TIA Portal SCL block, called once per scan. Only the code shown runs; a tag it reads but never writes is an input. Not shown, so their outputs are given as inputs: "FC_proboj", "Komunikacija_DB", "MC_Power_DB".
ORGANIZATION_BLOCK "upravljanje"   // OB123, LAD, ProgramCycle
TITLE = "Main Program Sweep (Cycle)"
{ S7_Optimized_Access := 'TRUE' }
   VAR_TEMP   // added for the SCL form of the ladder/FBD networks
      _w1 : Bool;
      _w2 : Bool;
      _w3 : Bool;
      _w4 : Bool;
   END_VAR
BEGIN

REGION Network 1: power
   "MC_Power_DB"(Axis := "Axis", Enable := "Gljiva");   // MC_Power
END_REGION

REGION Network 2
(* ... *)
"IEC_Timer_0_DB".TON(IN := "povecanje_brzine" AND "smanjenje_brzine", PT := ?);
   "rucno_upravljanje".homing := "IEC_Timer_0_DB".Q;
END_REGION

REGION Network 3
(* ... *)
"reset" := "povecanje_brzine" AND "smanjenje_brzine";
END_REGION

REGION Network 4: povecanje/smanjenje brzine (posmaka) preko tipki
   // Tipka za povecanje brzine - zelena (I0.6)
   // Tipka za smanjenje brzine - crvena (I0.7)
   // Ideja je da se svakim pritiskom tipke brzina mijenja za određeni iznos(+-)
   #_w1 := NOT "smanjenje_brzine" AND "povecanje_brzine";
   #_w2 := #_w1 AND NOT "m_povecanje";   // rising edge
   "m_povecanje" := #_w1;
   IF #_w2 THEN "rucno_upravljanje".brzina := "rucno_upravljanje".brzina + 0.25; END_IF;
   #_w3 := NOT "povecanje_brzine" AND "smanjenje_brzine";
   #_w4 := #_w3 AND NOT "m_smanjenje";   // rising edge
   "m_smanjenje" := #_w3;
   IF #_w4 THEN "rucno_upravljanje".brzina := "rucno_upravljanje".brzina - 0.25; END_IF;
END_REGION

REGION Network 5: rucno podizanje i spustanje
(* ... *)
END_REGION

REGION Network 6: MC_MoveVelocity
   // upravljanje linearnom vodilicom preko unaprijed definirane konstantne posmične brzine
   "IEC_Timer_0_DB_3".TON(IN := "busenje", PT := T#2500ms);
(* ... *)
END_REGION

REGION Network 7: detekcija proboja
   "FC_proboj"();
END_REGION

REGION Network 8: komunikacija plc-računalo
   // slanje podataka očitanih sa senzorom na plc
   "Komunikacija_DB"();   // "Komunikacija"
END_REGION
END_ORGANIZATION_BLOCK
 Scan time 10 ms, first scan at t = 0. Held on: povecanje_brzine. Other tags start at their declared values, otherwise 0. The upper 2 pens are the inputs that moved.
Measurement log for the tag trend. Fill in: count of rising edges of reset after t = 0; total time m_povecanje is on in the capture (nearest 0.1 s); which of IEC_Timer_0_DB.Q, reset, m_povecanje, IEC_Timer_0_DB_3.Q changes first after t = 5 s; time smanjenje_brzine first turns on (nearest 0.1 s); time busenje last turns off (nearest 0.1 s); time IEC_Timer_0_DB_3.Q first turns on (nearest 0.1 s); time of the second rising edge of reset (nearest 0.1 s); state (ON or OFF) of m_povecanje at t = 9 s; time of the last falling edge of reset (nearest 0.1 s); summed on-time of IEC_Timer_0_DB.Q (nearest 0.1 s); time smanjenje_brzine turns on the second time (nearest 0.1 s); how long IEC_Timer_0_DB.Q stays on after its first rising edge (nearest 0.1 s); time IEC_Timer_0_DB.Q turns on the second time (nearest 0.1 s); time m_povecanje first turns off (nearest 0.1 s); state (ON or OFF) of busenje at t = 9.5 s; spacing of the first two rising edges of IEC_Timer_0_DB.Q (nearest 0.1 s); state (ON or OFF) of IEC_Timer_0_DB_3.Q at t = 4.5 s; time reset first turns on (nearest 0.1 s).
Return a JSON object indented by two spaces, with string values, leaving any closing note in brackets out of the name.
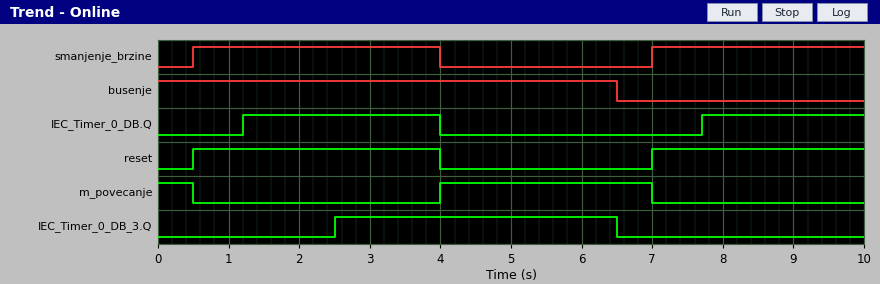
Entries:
{
  "count of rising edges of reset after t = 0": "2",
  "total time m_povecanje is on in the capture": "3.5 s",
  "which of IEC_Timer_0_DB.Q, reset, m_povecanje, IEC_Timer_0_DB_3.Q changes first after t = 5 s": "IEC_Timer_0_DB_3.Q",
  "time smanjenje_brzine first turns on": "0.5 s",
  "time busenje last turns off": "6.5 s",
  "time IEC_Timer_0_DB_3.Q first turns on": "2.5 s",
  "time of the second rising edge of reset": "7.0 s",
  "state (ON or OFF) of m_povecanje at t = 9 s": "OFF",
  "time of the last falling edge of reset": "4.0 s",
  "summed on-time of IEC_Timer_0_DB.Q": "5.1 s",
  "time smanjenje_brzine turns on the second time": "7.0 s",
  "how long IEC_Timer_0_DB.Q stays on after its first rising edge": "2.8 s",
  "time IEC_Timer_0_DB.Q turns on the second time": "7.7 s",
  "time m_povecanje first turns off": "0.5 s",
  "state (ON or OFF) of busenje at t = 9.5 s": "OFF",
  "spacing of the first two rising edges of IEC_Timer_0_DB.Q": "6.5 s",
  "state (ON or OFF) of IEC_Timer_0_DB_3.Q at t = 4.5 s": "ON",
  "time reset first turns on": "0.5 s"
}
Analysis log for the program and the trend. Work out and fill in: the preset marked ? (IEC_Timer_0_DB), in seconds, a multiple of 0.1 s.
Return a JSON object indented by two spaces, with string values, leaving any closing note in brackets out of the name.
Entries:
{
  "the preset marked ? (IEC_Timer_0_DB), in seconds, a multiple of 0.1 s": "0.7 s"
}
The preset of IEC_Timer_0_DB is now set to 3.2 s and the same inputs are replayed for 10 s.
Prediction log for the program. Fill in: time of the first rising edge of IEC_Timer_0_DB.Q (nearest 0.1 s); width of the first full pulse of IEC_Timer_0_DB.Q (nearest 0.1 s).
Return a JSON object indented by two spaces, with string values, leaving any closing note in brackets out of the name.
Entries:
{
  "time of the first rising edge of IEC_Timer_0_DB.Q": "3.7 s",
  "width of the first full pulse of IEC_Timer_0_DB.Q": "0.3 s"
}
